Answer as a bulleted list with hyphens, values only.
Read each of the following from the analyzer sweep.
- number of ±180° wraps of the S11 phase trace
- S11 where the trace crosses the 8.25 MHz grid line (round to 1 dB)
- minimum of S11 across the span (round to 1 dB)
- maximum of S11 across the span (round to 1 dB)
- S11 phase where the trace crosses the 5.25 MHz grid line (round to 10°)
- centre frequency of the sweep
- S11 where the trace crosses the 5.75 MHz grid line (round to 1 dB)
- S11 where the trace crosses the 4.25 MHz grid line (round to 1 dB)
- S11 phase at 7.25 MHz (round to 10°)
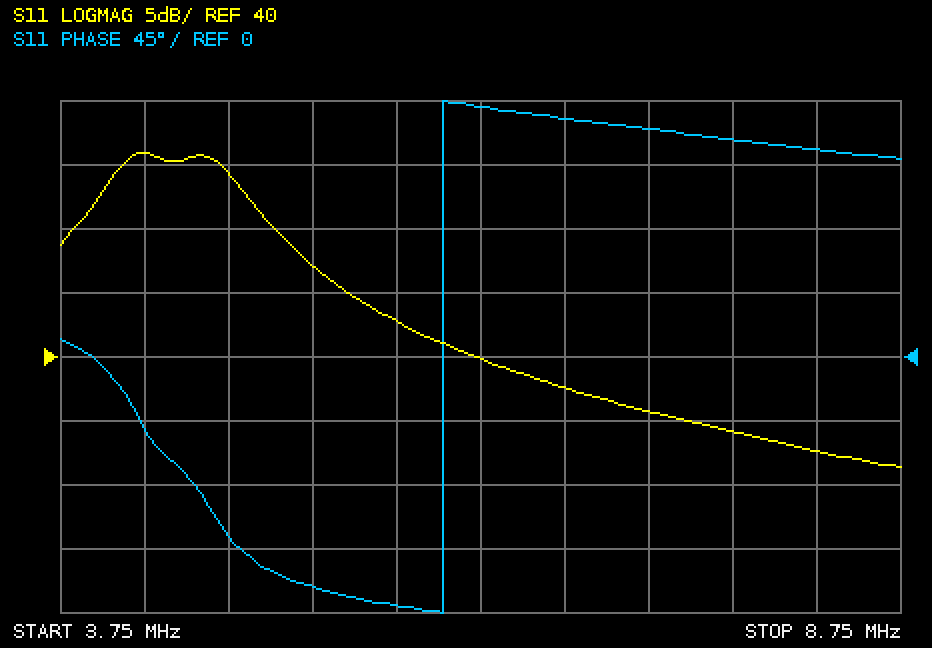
- 1
- 33 dB
- 31 dB
- 56 dB
- -160°
- 6.25 MHz
- 43 dB
- 56 dB
- 160°
